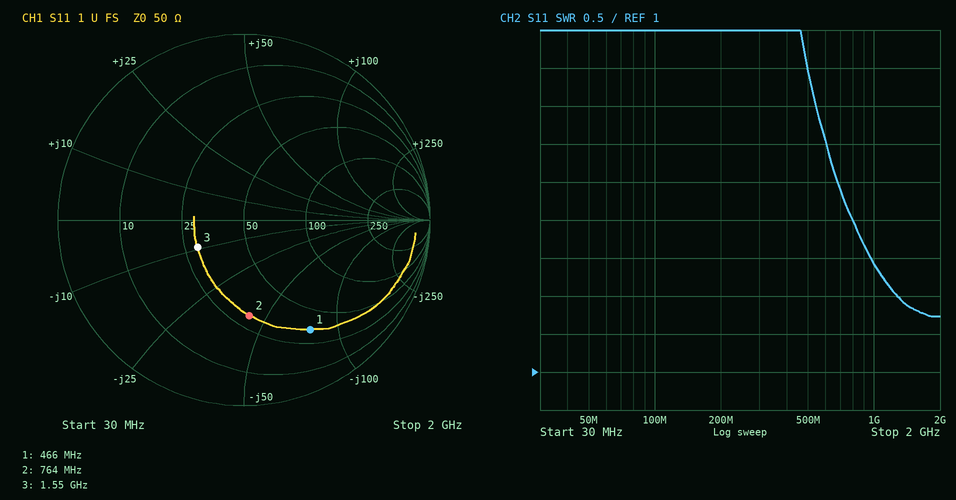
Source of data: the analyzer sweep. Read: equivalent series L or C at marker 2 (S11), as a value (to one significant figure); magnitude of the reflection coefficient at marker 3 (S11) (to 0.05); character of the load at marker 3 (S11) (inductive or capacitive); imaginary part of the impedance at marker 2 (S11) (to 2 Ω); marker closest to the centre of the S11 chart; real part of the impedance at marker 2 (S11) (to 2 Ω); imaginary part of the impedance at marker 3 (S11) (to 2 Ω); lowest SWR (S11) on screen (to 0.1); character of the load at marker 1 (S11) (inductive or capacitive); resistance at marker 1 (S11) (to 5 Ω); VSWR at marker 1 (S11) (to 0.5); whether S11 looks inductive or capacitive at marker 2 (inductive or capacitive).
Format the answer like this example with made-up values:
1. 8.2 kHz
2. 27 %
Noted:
1. 5 pF
2. 0.30
3. capacitive
4. -42 Ω
5. marker 3
6. 30 Ω
7. -10 Ω
8. 1.7
9. capacitive
10. 35 Ω
11. 5.5
12. capacitive
